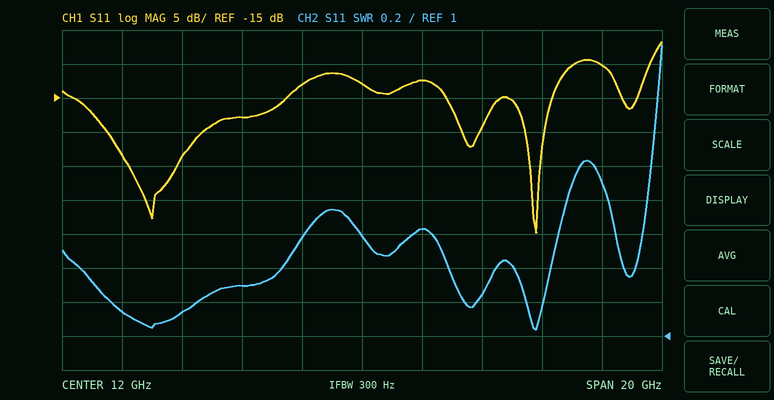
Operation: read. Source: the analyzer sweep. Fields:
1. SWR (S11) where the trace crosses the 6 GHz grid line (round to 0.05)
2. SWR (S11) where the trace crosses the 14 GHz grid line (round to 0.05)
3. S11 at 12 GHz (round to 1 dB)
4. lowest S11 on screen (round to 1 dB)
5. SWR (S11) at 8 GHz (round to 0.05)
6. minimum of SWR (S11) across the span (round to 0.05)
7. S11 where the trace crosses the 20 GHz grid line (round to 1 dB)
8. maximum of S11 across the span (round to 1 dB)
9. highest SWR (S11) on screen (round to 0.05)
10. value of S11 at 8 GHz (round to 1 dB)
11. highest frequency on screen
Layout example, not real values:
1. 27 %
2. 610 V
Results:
1. 1.15
2. 1.65
3. -13 dB
4. -35 dB
5. 1.30
6. 1.05
7. -10 dB
8. -7 dB
9. 2.70
10. -18 dB
11. 22 GHz
